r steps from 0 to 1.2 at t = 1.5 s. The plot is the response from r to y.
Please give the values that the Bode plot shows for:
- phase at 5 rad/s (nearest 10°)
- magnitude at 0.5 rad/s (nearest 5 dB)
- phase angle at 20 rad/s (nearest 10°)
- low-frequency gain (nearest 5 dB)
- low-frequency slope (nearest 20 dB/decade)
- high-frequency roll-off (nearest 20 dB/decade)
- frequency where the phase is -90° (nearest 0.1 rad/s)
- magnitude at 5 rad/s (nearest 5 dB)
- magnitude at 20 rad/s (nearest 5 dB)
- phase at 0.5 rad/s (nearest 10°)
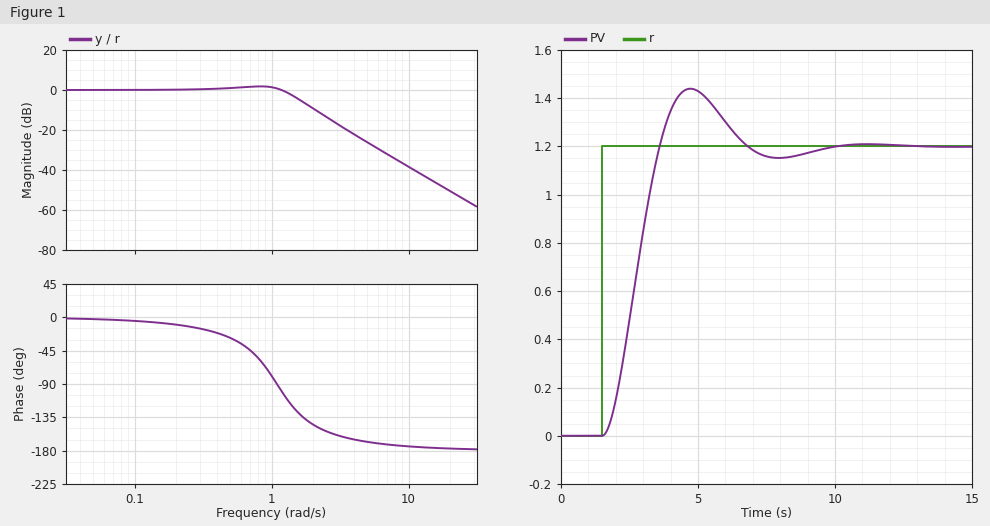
-170°
0 dB
-180°
0 dB
0 dB/decade
-40 dB/decade
1.1 rad/s
-25 dB
-50 dB
-30°
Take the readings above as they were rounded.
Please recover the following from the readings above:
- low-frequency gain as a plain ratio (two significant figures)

1.0
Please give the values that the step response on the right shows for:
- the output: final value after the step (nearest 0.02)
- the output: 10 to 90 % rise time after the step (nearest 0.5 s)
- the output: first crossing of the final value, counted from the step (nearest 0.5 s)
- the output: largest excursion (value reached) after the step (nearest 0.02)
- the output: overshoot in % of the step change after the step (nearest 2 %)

1.20
1.5 s
2.0 s
1.44
20 %
